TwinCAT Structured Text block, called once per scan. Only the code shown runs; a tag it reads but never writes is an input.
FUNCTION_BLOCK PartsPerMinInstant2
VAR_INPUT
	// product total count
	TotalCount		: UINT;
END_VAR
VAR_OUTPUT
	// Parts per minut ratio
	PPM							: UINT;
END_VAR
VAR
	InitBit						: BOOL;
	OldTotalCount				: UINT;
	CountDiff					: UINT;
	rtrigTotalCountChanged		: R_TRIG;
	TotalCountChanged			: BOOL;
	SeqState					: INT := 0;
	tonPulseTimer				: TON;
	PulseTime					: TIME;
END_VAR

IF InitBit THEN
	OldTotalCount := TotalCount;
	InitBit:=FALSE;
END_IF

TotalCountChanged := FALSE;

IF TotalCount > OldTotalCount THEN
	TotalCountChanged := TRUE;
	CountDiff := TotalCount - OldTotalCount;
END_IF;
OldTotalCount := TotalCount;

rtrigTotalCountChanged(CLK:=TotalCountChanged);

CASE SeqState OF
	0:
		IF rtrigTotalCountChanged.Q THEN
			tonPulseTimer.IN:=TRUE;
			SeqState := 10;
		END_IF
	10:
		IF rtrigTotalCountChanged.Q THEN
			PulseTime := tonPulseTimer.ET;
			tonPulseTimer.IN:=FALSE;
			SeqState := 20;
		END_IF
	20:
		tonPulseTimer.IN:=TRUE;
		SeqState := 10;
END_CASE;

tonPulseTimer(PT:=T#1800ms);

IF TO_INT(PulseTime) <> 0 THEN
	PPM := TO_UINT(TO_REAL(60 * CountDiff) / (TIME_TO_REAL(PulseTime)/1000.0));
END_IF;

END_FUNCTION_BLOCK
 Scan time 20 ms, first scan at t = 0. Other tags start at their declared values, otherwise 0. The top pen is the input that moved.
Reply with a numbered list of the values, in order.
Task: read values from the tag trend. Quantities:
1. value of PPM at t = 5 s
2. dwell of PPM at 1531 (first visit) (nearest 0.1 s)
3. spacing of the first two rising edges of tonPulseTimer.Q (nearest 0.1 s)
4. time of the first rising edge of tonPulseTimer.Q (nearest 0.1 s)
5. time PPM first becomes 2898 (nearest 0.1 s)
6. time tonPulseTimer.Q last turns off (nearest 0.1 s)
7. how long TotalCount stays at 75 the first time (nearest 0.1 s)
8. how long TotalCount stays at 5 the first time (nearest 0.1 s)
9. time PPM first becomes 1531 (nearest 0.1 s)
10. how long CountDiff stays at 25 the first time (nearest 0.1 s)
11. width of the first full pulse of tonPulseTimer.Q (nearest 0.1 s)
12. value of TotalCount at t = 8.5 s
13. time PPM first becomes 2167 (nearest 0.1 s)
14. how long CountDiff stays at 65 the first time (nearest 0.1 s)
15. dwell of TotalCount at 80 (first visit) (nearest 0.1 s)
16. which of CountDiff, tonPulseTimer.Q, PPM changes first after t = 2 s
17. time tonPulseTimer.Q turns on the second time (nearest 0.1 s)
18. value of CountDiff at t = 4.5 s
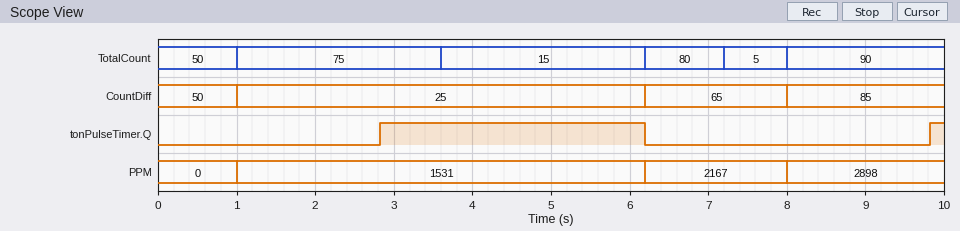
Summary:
1. 1531
2. 5.2 s
3. 7.0 s
4. 2.8 s
5. 8.0 s
6. 6.2 s
7. 2.6 s
8. 0.8 s
9. 1.0 s
10. 5.2 s
11. 3.4 s
12. 90
13. 6.2 s
14. 1.8 s
15. 1.0 s
16. tonPulseTimer.Q
17. 9.8 s
18. 25
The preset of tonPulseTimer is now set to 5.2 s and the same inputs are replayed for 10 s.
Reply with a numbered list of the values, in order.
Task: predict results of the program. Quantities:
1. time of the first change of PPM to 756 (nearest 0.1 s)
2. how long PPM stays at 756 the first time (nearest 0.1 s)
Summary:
1. 6.2 s
2. 1.8 s
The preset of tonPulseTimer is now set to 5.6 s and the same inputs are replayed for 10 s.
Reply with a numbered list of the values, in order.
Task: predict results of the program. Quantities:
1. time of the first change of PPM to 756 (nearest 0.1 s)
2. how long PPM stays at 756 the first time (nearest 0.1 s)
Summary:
1. 6.2 s
2. 1.8 s
